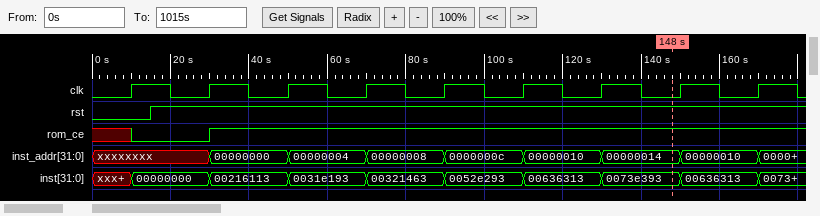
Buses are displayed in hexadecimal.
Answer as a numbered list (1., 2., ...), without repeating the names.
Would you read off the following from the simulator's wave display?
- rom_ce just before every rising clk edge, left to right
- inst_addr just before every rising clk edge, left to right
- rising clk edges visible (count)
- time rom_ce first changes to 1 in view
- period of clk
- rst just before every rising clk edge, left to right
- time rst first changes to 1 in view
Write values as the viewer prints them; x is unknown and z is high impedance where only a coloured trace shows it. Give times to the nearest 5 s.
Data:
1. x 0 1 1 1 1 1 1 1
2. xxxxxxxx, xxxxxxxx, 00000000, 00000004, 00000008, 0000000c, 00000010, 00000014, 00000010
3. 9
4. 30 s
5. 20 s
6. 0 1 1 1 1 1 1 1 1
7. 15 s
